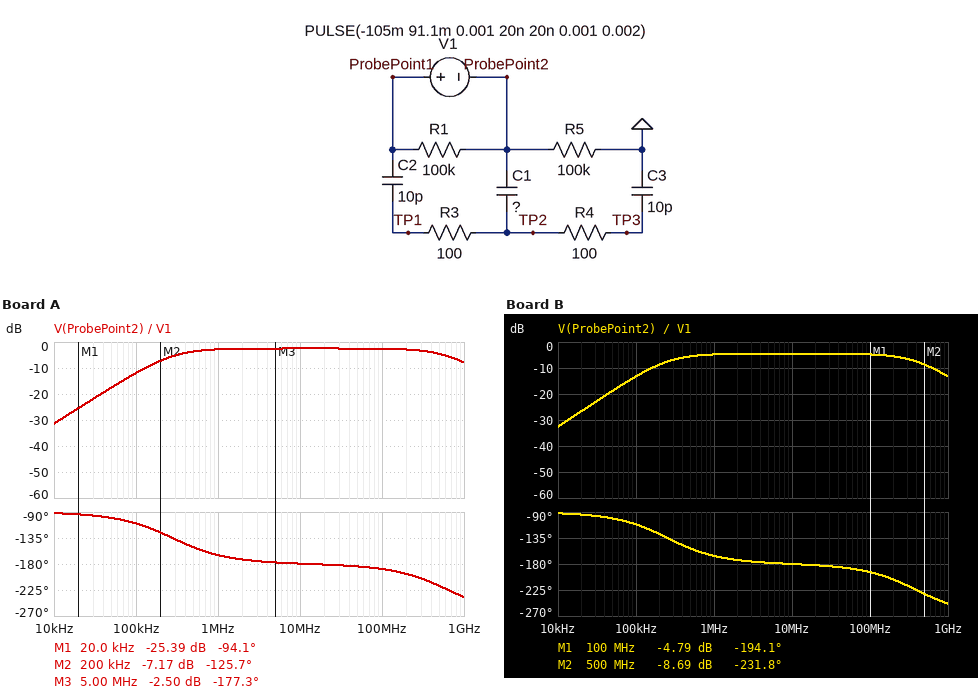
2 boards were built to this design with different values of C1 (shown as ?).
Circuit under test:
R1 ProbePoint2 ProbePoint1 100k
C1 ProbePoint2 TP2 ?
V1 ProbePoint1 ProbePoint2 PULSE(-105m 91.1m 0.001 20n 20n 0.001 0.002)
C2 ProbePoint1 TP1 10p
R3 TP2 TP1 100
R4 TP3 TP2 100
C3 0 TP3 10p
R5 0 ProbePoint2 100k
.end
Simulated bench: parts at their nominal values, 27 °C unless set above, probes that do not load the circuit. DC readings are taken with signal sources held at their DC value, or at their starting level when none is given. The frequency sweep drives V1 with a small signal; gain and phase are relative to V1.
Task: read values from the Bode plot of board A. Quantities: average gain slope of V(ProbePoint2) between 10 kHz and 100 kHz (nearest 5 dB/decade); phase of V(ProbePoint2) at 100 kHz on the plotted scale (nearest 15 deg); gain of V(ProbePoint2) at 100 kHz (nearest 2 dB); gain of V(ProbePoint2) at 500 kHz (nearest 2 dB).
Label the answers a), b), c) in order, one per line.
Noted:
a) 20 dB/decade
b) -105 deg
c) -12 dB
d) -4 dB
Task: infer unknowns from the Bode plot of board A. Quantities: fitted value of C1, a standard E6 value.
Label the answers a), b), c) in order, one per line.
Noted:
a) 3.3 pF
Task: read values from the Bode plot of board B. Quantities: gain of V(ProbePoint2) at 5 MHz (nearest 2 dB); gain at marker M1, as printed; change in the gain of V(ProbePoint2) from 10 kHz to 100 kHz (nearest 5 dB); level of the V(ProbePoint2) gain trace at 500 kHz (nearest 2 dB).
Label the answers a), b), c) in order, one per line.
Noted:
a) -4 dB
b) -4.79 dB
c) 20 dB
d) -6 dB
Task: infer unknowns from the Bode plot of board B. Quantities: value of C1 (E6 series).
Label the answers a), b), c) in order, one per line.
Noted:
a) 6.8 pF
